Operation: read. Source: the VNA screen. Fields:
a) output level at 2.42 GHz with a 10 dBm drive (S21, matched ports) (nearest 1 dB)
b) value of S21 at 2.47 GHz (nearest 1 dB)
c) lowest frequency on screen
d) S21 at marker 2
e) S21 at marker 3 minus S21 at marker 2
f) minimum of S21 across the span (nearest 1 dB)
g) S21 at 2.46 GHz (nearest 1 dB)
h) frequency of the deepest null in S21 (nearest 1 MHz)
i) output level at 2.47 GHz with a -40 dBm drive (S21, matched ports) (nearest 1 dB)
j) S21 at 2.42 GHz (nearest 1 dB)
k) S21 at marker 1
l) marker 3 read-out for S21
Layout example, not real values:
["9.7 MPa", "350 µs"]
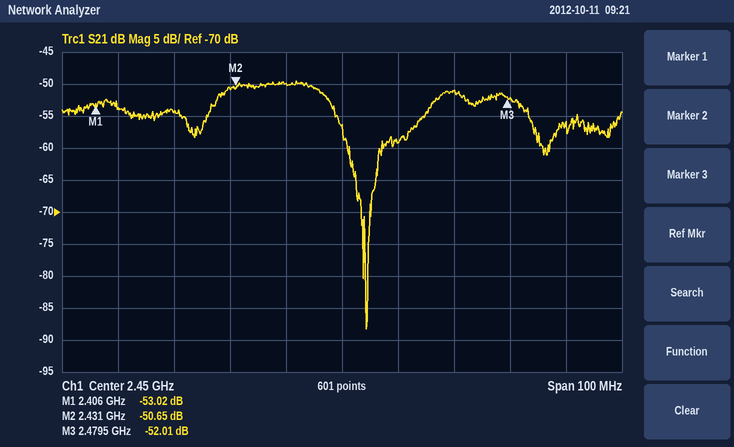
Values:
["-44 dBm", "-51 dB", "2.4 GHz", "-50.65 dB", "-1.36 dB", "-88 dB", "-59 dB", "2.454 GHz", "-91 dBm", "-54 dB", "-53.02 dB", "-52.01 dB"]
